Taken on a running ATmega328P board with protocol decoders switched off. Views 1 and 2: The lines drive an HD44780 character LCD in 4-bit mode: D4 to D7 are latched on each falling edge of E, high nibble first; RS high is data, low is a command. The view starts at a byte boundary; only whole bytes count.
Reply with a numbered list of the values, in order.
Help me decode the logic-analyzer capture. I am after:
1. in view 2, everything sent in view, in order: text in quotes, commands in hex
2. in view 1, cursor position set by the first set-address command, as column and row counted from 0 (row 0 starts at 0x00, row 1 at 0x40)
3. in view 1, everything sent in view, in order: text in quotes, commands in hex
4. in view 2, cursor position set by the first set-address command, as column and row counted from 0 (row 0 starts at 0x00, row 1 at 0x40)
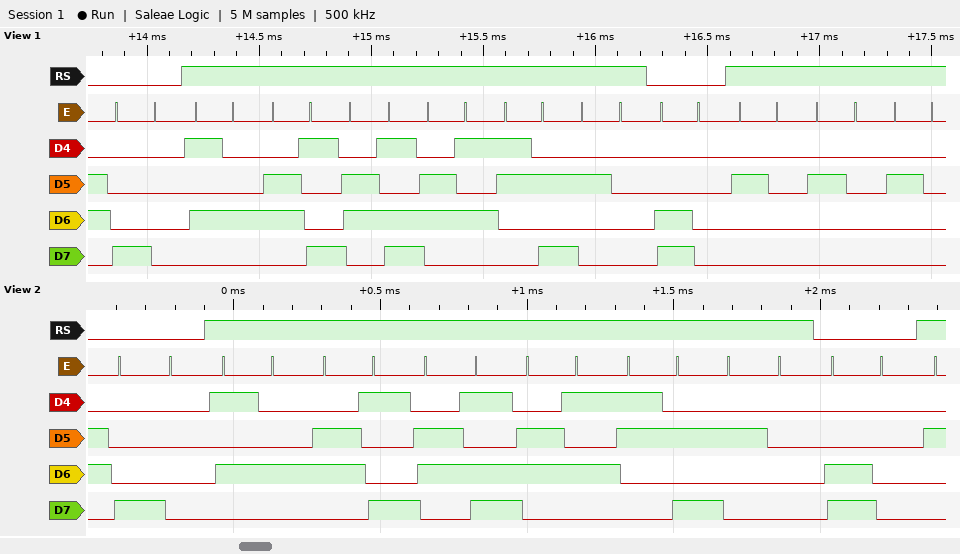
1. 0x80 "Time: " 0xC0
2. column 0, row 0
3. 0x80 "Time: " 0xC0 "   "
4. column 0, row 0
